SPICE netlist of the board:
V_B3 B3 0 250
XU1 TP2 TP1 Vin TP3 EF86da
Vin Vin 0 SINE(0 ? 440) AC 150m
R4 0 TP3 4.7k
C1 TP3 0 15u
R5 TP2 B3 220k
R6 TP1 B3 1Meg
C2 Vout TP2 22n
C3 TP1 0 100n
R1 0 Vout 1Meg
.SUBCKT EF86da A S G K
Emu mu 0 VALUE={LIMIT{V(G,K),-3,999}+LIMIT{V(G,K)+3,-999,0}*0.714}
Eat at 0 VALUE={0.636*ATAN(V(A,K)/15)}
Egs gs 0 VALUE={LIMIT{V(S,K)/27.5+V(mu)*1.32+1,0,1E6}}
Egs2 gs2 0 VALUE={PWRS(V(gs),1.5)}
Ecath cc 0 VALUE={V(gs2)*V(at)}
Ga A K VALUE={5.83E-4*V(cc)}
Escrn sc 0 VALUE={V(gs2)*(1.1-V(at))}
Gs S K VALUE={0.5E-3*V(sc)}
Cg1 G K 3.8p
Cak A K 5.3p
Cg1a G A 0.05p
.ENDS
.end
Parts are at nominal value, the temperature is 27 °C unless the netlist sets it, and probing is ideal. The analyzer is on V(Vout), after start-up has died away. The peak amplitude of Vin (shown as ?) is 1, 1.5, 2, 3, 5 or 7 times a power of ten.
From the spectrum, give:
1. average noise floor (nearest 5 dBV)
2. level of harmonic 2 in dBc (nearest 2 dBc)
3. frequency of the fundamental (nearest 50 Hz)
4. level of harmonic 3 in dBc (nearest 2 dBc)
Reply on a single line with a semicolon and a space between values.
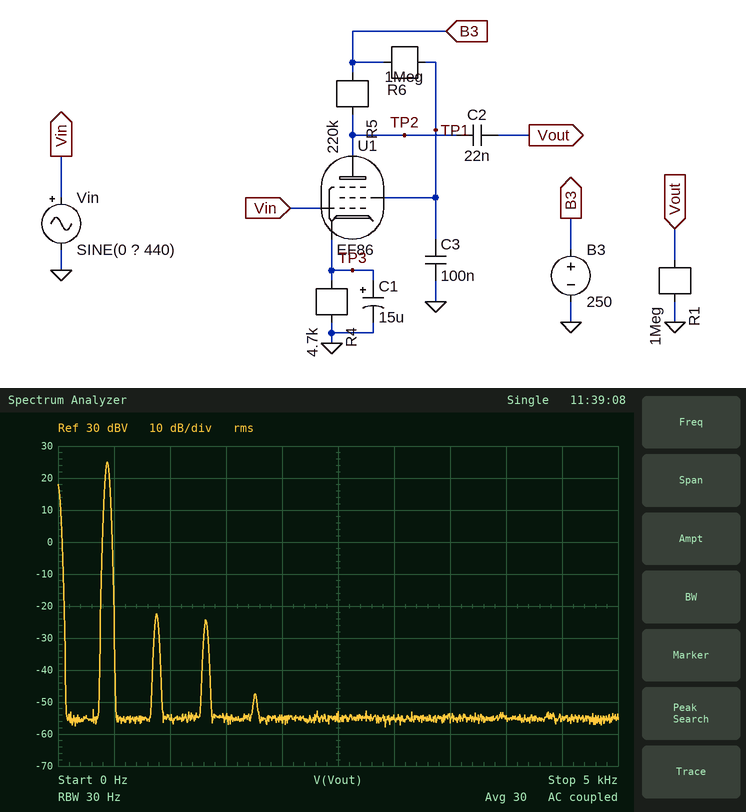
-55 dBV; -48 dBc; 450 Hz; -50 dBc
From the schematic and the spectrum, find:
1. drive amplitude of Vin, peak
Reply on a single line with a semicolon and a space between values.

200 mV
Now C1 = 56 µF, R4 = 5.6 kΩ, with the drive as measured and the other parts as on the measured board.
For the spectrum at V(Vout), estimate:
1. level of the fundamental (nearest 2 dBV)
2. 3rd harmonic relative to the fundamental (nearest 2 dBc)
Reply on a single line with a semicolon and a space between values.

26 dBV; -50 dBc
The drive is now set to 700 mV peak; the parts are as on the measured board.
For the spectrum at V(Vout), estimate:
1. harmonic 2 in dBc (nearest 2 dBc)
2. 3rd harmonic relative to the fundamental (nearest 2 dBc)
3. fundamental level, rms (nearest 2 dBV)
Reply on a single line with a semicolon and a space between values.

-22 dBc; -30 dBc; 36 dBV
